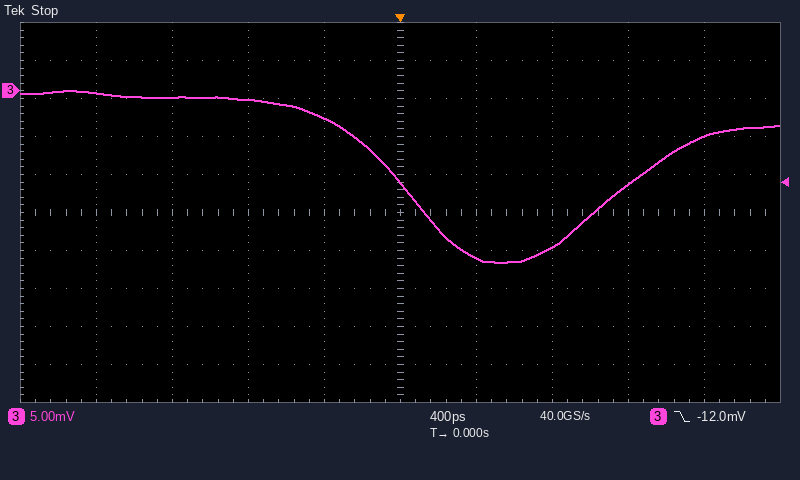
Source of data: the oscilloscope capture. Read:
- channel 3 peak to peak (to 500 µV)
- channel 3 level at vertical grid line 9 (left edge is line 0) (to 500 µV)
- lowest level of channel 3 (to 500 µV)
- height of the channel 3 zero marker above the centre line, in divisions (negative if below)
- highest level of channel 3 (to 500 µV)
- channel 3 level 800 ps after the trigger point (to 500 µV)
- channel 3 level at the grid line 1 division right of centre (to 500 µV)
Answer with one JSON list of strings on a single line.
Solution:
["22.5 mV", "-6.0 mV", "-22.5 mV", "+3.2 div", "0.0 mV", "-20.5 mV", "-22.0 mV"]
